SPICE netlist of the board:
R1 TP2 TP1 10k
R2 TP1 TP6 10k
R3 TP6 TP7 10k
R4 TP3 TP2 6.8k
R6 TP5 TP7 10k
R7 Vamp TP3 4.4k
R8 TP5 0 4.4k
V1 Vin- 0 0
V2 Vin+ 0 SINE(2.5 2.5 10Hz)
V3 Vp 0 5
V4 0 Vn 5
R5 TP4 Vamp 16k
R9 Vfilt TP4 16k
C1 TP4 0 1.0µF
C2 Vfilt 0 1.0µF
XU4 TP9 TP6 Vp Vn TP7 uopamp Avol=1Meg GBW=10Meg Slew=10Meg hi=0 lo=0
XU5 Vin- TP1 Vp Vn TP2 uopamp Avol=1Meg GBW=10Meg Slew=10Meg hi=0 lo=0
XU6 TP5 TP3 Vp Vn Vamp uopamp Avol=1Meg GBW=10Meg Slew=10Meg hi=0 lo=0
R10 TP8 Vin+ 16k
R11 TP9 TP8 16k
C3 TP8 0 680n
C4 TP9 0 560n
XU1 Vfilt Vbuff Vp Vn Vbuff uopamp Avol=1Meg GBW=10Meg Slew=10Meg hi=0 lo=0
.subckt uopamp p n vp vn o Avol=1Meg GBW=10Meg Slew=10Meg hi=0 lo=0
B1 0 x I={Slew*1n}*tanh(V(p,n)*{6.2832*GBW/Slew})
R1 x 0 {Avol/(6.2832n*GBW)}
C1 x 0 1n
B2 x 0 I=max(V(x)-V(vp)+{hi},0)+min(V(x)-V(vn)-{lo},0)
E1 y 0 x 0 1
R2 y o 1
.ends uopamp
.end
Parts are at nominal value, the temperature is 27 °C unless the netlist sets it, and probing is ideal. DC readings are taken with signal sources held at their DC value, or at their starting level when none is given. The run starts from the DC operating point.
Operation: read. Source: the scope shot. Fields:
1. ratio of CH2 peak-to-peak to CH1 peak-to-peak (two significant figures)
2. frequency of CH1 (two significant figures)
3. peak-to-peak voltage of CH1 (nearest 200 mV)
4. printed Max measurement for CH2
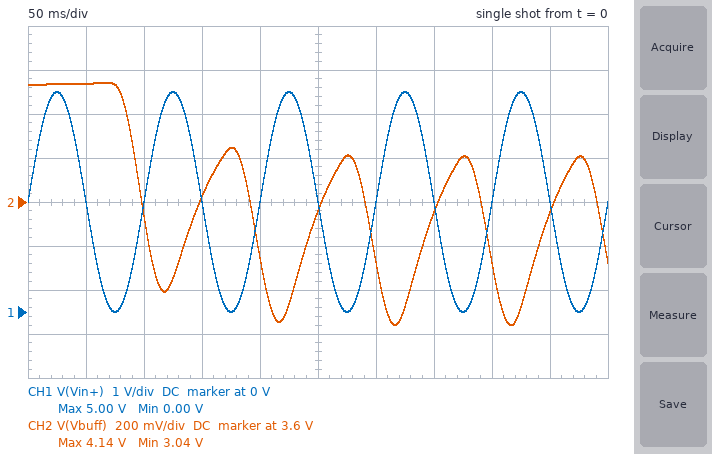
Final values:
0.22
10 Hz
5.0 V
4.14 V
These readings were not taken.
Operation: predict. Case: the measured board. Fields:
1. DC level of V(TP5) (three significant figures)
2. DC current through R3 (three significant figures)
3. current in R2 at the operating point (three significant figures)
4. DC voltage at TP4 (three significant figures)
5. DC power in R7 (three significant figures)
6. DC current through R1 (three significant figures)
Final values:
1.53 V
250 µA
250 µA
4.13 V
1.54 mW
250 µA
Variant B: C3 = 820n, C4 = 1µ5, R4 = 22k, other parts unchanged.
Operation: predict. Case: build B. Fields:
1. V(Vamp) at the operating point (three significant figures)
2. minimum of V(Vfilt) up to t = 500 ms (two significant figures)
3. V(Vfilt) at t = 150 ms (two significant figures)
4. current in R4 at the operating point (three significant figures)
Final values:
2.33 V
2.0 V
2.2 V
183 µA
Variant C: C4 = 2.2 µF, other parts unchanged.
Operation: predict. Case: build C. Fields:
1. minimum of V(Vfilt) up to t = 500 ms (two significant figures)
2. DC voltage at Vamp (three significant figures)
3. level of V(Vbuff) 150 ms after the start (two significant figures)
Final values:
3.7 V
4.13 V
4.0 V
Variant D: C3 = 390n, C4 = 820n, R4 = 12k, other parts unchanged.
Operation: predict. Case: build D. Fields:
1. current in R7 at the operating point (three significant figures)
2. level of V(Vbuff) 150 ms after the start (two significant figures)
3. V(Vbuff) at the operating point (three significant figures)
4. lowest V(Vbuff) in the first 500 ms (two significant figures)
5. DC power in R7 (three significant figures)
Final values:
336 µA
2.7 V
3.00 V
2.3 V
496 µW
